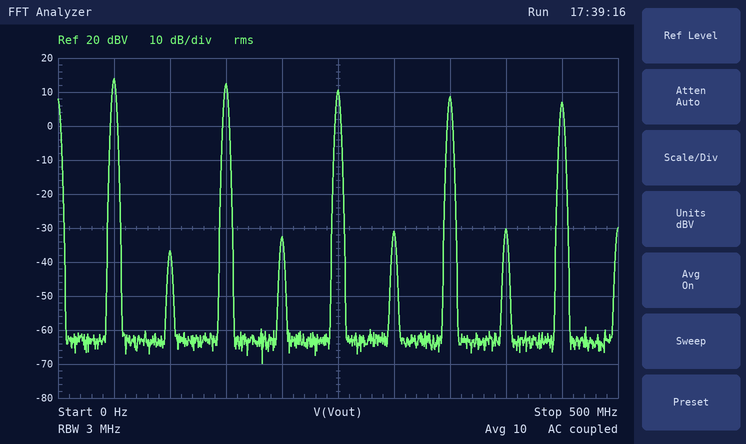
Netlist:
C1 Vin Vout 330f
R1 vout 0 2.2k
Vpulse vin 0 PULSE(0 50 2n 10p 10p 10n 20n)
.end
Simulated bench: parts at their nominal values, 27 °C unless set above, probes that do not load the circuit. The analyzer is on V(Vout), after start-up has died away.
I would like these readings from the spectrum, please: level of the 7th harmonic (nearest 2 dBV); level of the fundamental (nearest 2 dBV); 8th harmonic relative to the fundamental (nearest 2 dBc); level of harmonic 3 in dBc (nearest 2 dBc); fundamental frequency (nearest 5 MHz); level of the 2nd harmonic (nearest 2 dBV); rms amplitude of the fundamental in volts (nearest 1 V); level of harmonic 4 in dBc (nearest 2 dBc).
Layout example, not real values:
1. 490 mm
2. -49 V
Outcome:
1. 8 dBV
2. 14 dBV
3. -44 dBc
4. -2 dBc
5. 50 MHz
6. -36 dBV
7. 5 V
8. -46 dBc
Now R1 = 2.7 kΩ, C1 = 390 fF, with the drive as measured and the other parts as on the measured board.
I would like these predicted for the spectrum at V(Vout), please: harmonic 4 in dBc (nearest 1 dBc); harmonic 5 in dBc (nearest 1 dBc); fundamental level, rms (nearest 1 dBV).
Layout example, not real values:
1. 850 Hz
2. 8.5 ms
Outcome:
1. -48 dBc
2. -5 dBc
3. 17 dBV
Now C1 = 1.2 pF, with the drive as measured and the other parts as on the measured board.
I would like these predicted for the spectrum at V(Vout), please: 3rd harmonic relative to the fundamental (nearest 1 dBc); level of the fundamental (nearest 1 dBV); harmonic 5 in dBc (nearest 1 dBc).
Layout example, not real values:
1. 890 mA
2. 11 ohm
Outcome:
1. -6 dBc
2. 23 dBV
3. -10 dBc
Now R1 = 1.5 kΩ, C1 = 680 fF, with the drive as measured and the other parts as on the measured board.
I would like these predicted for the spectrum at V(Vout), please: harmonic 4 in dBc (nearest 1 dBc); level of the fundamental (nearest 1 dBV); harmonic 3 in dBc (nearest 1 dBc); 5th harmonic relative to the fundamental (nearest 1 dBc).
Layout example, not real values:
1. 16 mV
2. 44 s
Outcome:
1. -48 dBc
2. 17 dBV
3. -2 dBc
4. -5 dBc
